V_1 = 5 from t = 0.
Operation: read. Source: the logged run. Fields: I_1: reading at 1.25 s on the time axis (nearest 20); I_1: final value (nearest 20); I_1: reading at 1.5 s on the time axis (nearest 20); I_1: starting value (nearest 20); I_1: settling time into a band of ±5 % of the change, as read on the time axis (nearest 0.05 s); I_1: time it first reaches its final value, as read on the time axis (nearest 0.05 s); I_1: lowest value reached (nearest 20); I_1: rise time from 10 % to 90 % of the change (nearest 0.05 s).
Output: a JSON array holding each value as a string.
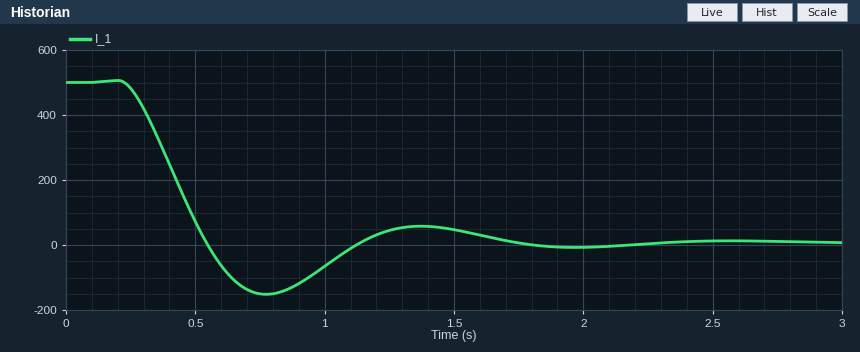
["40", "0", "40", "500", "1.60 s", "0.55 s", "-160", "0.25 s"]
